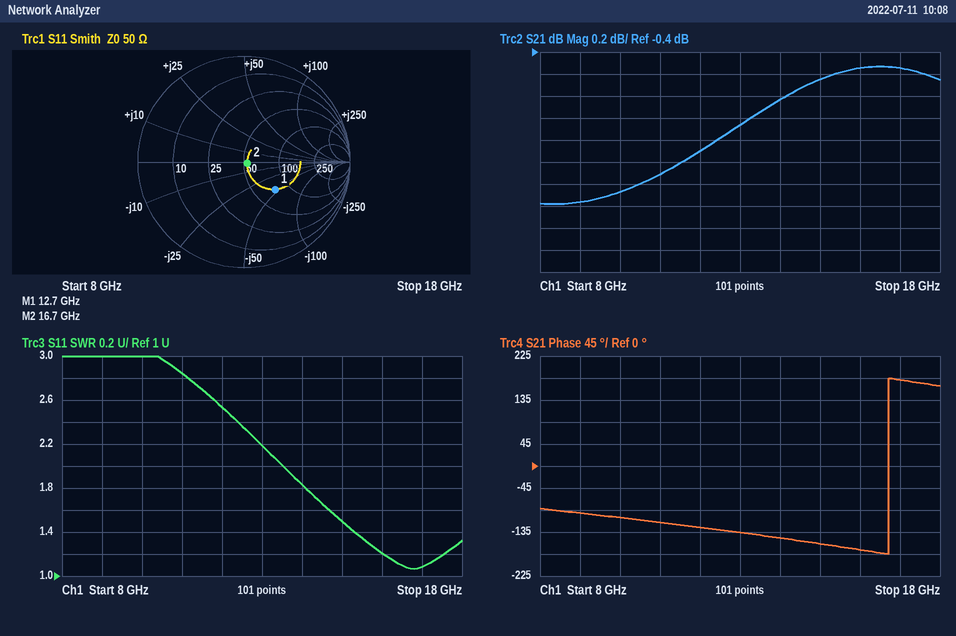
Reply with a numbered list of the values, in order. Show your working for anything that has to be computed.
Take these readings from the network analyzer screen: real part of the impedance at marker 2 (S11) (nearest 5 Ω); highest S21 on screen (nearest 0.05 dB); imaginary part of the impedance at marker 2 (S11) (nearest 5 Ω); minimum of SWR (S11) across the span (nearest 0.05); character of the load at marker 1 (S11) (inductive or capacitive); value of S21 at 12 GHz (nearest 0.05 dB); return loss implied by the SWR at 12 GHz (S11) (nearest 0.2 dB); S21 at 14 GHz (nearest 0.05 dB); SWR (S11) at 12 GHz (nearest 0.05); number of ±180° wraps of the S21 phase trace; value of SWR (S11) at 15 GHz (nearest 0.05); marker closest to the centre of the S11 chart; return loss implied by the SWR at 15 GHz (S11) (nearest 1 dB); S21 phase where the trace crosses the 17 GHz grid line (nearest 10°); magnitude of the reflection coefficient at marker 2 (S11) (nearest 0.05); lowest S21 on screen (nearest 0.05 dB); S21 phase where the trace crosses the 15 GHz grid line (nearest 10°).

1. 55 Ω
2. -0.55 dB
3. 0 Ω
4. 1.05
5. capacitive
6. -1.30 dB
7. −20 log10((2.55 − 1)/(2.55 + 1)) ≈ 7.2 dB
8. -0.85 dB
9. 2.55
10. 1
11. 1.50
12. marker 2
13. −20 log10((1.5 − 1)/(1.5 + 1)) ≈ 14 dB
14. 180°
15. 0.05
16. -1.80 dB
17. -160°
